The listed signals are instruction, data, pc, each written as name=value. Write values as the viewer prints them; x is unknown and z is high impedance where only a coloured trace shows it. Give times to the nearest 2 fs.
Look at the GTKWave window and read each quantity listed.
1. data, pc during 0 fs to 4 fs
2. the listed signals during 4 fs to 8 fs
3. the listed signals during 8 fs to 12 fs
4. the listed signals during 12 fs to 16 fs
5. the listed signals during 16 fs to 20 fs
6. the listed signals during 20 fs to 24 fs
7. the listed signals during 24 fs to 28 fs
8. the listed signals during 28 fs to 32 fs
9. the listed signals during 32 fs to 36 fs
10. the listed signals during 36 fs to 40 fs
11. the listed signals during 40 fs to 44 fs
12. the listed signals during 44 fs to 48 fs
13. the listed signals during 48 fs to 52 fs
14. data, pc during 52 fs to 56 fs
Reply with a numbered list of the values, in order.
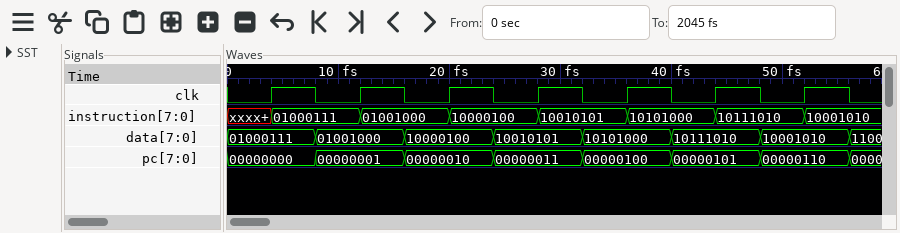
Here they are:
1. data=01000111, pc=00000000
2. instruction=01000111, data=01000111, pc=00000000
3. instruction=01000111, data=01001000, pc=00000001
4. instruction=01001000, data=01001000, pc=00000001
5. instruction=01001000, data=10000100, pc=00000010
6. instruction=10000100, data=10000100, pc=00000010
7. instruction=10000100, data=10010101, pc=00000011
8. instruction=10010101, data=10010101, pc=00000011
9. instruction=10010101, data=10101000, pc=00000100
10. instruction=10101000, data=10101000, pc=00000100
11. instruction=10101000, data=10111010, pc=00000101
12. instruction=10111010, data=10111010, pc=00000101
13. instruction=10111010, data=10001010, pc=00000110
14. data=10001010, pc=00000110
